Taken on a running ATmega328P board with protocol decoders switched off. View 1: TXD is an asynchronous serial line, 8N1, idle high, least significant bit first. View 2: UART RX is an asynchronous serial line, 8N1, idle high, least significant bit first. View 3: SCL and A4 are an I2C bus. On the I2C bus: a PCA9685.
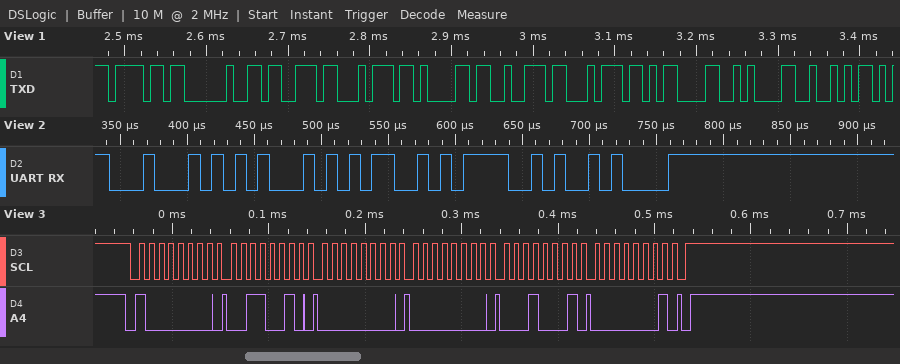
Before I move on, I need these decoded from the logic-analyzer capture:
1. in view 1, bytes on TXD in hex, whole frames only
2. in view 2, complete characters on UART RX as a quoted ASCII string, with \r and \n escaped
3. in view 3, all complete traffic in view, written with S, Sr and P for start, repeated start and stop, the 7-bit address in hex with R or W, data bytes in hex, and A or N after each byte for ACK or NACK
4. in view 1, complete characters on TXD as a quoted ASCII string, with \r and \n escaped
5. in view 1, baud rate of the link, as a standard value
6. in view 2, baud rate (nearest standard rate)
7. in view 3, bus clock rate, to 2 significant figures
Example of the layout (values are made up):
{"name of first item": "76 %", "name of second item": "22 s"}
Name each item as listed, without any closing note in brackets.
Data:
{"in view 1, bytes on TXD in hex, whole frames only": "0x6F 0x20 0x73 0x74 0x61 0x72 0x74 0x0D 0x0A 0x52", "in view 2, complete characters on UART RX as a quoted ASCII string, with \\r and \\n escaped": "\"DEMO\\n\"", "in view 3, all complete traffic in view, written with S, Sr and P for start, repeated start and stop, the 7-bit address in hex with R or W, data bytes in hex, and A or N after each byte for ACK or NACK": "S 40W A 32 A 00 A 00 A 11 A 01 A P", "in view 1, complete characters on TXD as a quoted ASCII string, with \\r and \\n escaped": "\"o start\\r\\nR\"", "in view 1, baud rate of the link, as a standard value": "115200 baud", "in view 2, baud rate": "115200 baud", "in view 3, bus clock rate, to 2 significant figures": "100 kHz"}
